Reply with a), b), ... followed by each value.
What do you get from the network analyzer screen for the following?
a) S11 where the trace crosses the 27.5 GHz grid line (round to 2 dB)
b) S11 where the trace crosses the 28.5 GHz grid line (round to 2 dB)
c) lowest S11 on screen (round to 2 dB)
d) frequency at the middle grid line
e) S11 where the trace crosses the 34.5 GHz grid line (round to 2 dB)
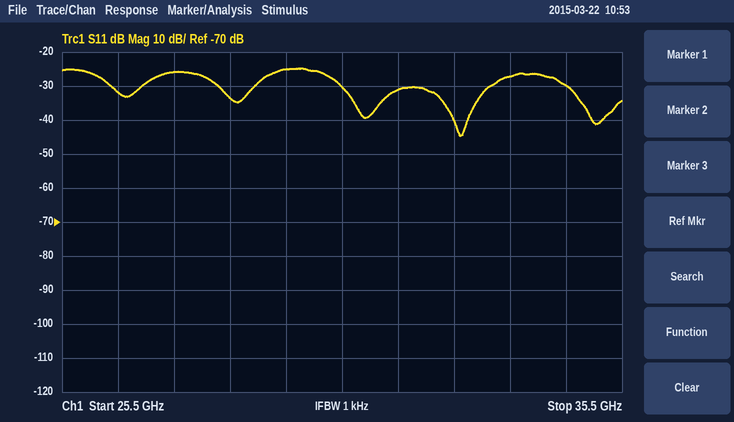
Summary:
a) -26 dB
b) -34 dB
c) -44 dB
d) 30.5 GHz
e) -30 dB
